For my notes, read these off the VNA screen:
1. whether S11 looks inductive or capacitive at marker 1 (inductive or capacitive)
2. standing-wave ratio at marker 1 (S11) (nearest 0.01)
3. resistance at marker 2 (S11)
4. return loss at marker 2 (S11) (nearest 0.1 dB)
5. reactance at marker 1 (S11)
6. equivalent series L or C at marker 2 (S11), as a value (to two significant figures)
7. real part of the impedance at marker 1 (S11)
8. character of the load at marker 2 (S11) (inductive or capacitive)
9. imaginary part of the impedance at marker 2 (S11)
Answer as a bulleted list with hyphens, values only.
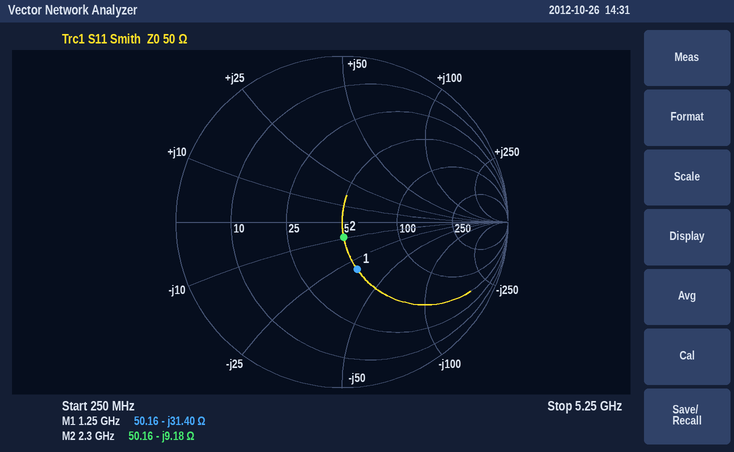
- capacitive
- 1.85
- 50.16 Ω
- 20.8 dB
- -31.40 Ω
- 7.5 pF
- 50.16 Ω
- capacitive
- -9.18 Ω
